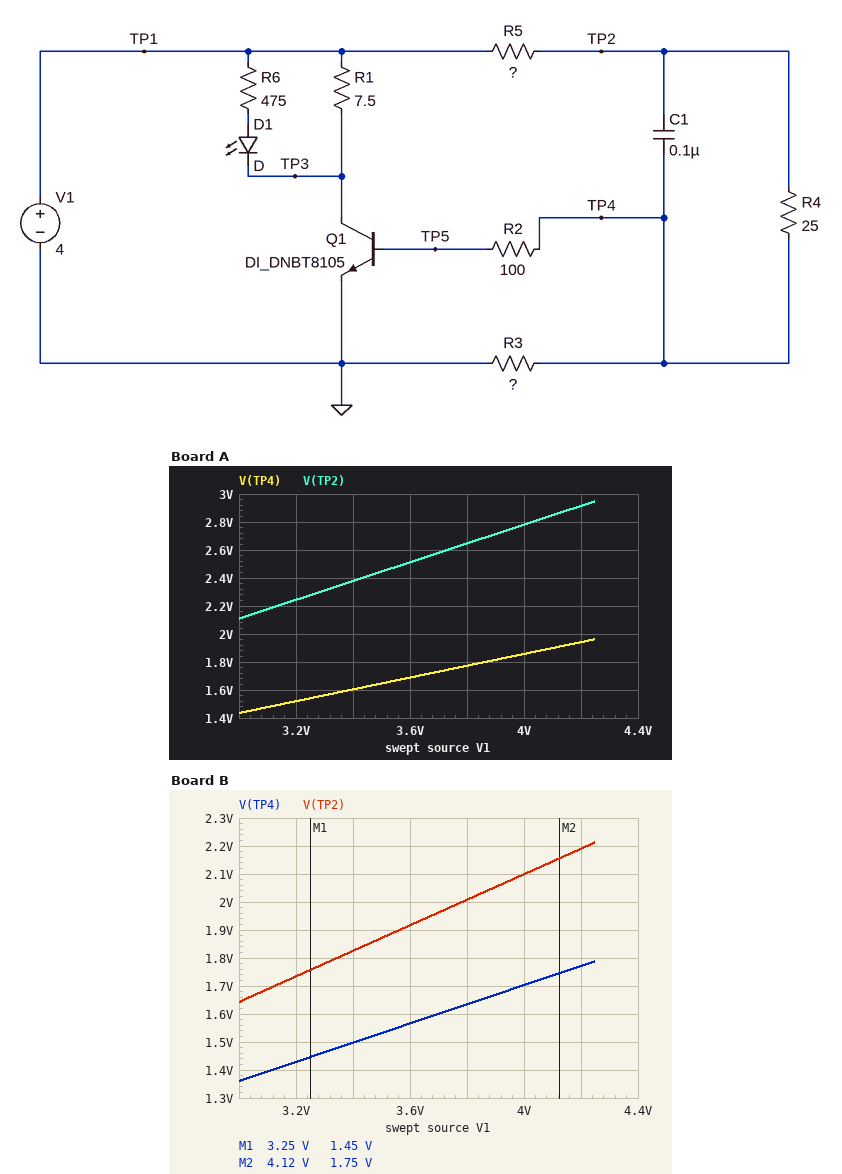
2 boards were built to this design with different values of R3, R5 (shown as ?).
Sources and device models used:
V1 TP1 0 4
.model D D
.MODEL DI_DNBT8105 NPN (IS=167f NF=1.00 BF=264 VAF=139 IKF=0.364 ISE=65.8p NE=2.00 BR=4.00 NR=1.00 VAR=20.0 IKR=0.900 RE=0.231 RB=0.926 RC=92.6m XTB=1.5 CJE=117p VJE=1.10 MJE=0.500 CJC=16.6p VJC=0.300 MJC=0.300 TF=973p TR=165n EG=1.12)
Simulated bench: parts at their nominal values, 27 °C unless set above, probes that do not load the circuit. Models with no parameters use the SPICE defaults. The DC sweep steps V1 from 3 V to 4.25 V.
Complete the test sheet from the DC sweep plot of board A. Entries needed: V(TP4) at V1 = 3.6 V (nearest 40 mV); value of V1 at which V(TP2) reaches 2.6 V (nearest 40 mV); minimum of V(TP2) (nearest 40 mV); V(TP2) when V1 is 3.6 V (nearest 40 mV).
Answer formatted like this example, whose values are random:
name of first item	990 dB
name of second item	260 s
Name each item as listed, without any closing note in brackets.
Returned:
V(TP4) at V1 = 3.6 V	1.68 V
value of V1 at which V(TP2) reaches 2.6 V	3.72 V
minimum of V(TP2)	2.12 V
V(TP2) when V1 is 3.6 V	2.52 V
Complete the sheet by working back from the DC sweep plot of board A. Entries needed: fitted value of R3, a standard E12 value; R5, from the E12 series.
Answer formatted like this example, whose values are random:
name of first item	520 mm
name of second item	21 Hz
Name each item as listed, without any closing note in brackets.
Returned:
fitted value of R3, a standard E12 value	68 Ω
R5, from the E12 series	33 Ω
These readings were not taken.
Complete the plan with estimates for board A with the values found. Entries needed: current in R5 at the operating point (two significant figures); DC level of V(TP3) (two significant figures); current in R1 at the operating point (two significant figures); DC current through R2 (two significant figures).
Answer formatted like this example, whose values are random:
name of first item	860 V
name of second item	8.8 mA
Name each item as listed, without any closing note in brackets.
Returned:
current in R5 at the operating point	37 mA
DC level of V(TP3)	280 mV
current in R1 at the operating point	500 mA
DC current through R2	9.6 mA
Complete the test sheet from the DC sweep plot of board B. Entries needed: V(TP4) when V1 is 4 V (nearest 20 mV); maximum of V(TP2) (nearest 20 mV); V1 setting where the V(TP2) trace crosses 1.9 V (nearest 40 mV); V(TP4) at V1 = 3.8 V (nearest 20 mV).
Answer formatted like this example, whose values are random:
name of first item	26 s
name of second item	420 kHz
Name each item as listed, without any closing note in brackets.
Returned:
V(TP4) when V1 is 4 V	1.70 V
maximum of V(TP2)	2.22 V
V1 setting where the V(TP2) trace crosses 1.9 V	3.56 V
V(TP4) at V1 = 3.8 V	1.64 V
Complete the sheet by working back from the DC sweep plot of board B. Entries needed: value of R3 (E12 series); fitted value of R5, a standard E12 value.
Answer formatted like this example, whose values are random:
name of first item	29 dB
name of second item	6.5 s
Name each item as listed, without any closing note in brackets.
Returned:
value of R3	220 Ω
fitted value of R5, a standard E12 value	120 Ω
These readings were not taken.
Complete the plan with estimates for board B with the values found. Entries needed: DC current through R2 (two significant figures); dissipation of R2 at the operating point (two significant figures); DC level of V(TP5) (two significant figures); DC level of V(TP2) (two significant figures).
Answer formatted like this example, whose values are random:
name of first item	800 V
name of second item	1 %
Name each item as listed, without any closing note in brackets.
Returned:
DC current through R2	8.1 mA
dissipation of R2 at the operating point	6.6 mW
DC level of V(TP5)	890 mV
DC level of V(TP2)	2.1 V
